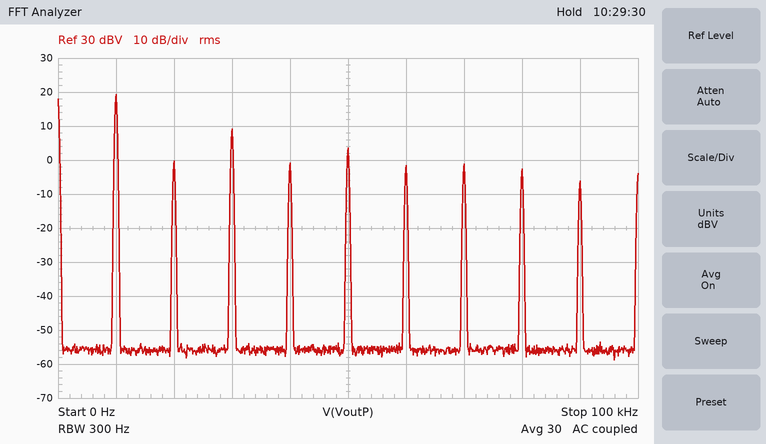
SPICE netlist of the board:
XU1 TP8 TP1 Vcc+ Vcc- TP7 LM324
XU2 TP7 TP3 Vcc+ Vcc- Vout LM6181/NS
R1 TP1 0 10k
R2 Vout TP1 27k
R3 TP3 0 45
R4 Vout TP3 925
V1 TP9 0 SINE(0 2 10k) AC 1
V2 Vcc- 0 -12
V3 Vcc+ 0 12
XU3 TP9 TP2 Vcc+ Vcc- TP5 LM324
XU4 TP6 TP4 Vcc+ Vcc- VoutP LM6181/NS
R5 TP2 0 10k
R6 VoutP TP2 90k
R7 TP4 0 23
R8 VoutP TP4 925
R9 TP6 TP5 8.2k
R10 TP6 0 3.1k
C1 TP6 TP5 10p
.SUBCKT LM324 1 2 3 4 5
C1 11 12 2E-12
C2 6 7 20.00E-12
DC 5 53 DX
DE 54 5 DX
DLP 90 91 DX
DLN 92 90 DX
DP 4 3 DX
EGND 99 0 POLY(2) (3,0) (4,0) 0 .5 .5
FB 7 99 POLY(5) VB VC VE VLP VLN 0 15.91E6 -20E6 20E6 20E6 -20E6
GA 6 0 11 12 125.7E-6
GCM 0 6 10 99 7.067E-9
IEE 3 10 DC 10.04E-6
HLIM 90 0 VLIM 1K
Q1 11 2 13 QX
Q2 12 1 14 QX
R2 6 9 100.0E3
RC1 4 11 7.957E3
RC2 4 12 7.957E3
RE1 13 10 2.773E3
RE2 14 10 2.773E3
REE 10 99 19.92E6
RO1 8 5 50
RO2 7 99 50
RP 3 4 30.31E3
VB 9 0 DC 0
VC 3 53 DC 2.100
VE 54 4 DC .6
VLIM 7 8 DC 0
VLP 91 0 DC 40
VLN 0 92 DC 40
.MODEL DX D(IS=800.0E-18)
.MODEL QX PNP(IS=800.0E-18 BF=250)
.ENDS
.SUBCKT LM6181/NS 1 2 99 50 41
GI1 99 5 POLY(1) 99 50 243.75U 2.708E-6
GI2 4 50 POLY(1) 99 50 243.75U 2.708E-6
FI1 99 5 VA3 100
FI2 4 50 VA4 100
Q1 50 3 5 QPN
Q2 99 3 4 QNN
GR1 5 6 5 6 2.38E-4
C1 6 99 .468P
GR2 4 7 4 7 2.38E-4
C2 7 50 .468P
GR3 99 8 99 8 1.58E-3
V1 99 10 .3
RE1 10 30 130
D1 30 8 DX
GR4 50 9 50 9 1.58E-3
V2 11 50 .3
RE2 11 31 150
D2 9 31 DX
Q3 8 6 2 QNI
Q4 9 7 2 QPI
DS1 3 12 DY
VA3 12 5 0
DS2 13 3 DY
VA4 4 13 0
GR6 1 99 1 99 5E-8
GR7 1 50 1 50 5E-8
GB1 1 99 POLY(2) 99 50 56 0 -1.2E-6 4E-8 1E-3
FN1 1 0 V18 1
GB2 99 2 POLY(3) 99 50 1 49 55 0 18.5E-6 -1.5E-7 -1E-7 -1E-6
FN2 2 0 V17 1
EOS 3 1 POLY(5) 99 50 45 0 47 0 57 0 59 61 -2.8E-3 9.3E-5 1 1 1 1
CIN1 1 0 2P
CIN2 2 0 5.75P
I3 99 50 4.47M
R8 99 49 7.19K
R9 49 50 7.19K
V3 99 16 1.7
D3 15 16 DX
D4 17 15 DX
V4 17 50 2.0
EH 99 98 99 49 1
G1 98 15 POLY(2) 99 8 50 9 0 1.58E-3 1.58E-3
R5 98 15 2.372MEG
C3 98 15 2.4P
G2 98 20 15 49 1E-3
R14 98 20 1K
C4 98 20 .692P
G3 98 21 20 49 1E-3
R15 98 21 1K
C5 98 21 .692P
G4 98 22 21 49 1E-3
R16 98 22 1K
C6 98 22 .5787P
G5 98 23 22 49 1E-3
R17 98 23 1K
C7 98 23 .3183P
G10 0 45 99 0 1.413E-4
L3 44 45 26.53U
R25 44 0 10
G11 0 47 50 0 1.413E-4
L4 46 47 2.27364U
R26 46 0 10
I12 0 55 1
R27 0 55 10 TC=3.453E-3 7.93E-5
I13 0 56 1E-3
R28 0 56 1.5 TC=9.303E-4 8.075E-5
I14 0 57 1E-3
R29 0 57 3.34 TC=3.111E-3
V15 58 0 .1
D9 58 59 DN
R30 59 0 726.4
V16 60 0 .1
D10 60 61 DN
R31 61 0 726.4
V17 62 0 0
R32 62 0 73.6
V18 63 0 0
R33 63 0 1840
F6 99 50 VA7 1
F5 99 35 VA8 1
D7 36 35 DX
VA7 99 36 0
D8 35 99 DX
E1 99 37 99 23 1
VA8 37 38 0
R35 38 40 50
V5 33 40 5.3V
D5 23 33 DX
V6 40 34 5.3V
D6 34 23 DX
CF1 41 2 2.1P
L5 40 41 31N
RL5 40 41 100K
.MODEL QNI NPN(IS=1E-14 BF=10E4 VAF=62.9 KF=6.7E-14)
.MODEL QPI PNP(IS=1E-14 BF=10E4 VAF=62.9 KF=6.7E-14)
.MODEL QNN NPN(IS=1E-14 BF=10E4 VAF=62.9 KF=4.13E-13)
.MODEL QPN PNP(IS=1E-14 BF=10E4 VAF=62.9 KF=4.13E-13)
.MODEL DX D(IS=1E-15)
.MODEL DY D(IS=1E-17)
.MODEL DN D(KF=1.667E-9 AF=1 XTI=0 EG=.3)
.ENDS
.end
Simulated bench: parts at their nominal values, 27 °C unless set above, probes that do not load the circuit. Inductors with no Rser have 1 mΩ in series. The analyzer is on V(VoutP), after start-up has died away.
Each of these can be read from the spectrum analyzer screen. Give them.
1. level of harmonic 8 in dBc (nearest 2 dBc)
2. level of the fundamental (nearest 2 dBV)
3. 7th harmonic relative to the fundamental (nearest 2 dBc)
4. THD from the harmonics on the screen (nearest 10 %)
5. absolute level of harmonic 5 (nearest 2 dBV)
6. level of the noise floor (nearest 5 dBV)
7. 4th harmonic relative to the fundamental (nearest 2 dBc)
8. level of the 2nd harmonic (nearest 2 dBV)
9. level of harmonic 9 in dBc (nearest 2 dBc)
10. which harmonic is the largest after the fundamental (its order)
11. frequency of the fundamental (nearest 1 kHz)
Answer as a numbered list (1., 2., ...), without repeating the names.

1. -22 dBc
2. 20 dBV
3. -20 dBc
4. 40 %
5. 4 dBV
6. -55 dBV
7. -20 dBc
8. 0 dBV
9. -26 dBc
10. 3
11. 10 kHz
